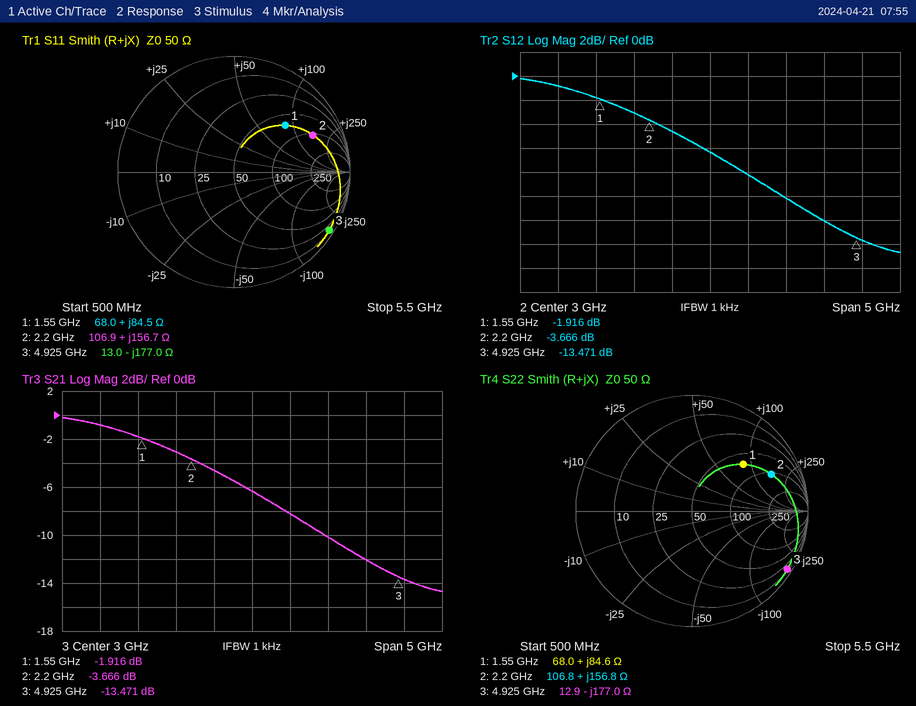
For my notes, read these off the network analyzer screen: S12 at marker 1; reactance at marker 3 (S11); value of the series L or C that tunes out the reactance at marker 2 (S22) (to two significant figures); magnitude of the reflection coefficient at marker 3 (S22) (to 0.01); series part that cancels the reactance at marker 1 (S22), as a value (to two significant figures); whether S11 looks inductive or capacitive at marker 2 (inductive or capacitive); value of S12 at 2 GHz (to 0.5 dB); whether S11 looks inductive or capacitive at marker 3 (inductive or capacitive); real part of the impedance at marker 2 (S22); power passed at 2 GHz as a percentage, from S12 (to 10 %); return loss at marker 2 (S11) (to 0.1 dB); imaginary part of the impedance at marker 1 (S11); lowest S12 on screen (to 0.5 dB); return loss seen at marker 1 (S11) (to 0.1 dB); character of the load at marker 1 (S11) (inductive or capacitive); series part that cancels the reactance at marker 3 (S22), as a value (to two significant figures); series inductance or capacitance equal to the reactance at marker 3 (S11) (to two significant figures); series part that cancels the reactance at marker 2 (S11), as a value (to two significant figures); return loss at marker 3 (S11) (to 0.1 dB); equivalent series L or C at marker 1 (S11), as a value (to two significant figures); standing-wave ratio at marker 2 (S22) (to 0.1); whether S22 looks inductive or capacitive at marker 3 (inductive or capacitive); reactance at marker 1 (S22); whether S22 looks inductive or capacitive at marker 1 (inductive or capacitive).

-1.916 dB
-177.0 Ω
460 fF
0.96
1.2 pF
inductive
-3.0 dB
capacitive
106.8 Ω
50 %
2.5 dB
+84.5 Ω
-14.5 dB
4.5 dB
inductive
5.7 nH
180 fF
460 fF
0.3 dB
8.7 nH
7.1
capacitive
+84.6 Ω
inductive
